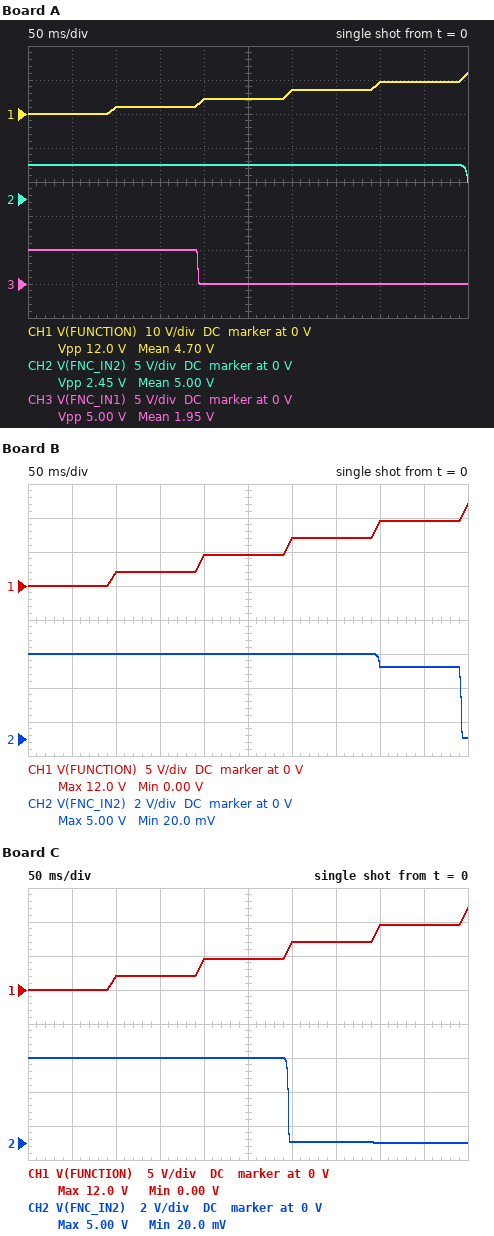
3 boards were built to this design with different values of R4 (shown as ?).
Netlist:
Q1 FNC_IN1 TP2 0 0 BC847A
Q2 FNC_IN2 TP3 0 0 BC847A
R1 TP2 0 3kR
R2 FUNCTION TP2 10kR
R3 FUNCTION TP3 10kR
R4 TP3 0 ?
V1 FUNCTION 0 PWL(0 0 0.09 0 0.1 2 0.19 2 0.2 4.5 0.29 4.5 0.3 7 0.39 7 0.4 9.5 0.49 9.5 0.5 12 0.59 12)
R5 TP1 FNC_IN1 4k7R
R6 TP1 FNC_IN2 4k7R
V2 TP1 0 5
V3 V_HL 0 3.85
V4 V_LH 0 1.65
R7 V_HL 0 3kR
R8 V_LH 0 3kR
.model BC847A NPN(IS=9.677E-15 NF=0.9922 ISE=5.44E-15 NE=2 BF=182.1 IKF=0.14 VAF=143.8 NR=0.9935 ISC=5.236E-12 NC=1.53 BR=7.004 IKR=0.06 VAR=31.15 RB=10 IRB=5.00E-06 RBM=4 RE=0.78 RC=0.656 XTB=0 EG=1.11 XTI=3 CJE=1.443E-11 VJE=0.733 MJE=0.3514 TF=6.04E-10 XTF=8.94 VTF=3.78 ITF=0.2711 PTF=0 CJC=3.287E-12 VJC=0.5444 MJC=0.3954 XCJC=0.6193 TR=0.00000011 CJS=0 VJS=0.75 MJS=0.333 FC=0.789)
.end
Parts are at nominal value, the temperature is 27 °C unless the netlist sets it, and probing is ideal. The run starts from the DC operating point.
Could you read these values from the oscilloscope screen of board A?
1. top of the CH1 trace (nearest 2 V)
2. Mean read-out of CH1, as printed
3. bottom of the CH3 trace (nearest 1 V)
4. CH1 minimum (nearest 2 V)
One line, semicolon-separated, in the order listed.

12 V; 4.70 V; 0 V; 0 V
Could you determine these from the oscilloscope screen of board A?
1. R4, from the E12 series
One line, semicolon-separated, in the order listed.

560 Ω
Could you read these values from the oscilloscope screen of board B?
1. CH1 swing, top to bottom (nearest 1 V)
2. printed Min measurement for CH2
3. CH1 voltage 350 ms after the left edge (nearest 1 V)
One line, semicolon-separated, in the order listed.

12 V; 20.0 mV; 7 V
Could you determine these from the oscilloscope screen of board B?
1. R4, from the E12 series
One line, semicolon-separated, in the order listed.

680 Ω
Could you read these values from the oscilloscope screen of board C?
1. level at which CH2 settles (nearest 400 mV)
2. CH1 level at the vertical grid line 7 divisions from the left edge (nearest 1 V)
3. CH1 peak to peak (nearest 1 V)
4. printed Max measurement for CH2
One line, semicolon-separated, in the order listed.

0 V; 7 V; 12 V; 5.00 V
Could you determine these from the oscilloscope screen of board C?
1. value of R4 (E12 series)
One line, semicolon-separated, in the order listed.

1.2 kΩ
